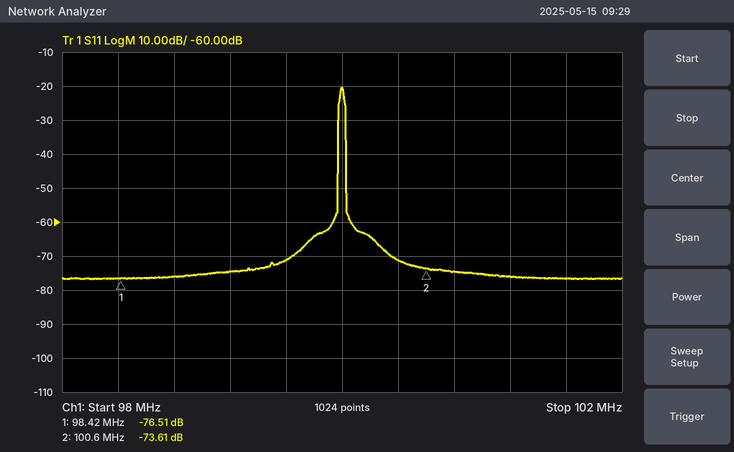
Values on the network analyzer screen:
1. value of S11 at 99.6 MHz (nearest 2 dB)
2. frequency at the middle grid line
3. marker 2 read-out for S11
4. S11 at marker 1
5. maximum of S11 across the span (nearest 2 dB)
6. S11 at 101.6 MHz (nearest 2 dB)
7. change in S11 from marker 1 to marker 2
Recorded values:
-72 dB
100 MHz
-73.61 dB
-76.51 dB
-20 dB
-76 dB
2.90 dB
